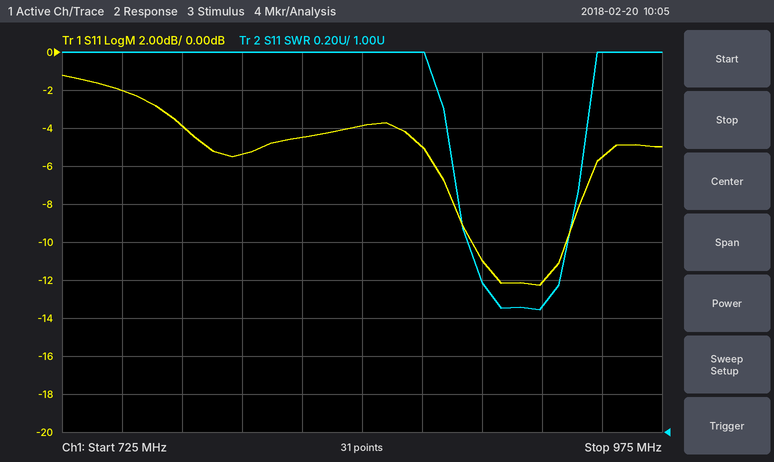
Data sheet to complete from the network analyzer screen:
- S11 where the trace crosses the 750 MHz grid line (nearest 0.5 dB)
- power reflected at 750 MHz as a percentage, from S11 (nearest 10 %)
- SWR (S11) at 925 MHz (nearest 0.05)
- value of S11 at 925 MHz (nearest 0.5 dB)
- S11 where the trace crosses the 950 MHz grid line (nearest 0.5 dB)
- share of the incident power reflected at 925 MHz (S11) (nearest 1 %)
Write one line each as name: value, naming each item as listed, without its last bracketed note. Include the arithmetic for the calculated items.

S11 where the trace crosses the 750 MHz grid line: -2.0 dB
power reflected at 750 MHz as a percentage, from S11: 10^(-2/10) ≈ 63.1 %, so 60 % to the nearest 10 %
SWR (S11) at 925 MHz: 1.65
value of S11 at 925 MHz: -12.0 dB
S11 where the trace crosses the 950 MHz grid line: -5.5 dB
share of the incident power reflected at 925 MHz (S11): 10^(-12/10) ≈ 6 %
